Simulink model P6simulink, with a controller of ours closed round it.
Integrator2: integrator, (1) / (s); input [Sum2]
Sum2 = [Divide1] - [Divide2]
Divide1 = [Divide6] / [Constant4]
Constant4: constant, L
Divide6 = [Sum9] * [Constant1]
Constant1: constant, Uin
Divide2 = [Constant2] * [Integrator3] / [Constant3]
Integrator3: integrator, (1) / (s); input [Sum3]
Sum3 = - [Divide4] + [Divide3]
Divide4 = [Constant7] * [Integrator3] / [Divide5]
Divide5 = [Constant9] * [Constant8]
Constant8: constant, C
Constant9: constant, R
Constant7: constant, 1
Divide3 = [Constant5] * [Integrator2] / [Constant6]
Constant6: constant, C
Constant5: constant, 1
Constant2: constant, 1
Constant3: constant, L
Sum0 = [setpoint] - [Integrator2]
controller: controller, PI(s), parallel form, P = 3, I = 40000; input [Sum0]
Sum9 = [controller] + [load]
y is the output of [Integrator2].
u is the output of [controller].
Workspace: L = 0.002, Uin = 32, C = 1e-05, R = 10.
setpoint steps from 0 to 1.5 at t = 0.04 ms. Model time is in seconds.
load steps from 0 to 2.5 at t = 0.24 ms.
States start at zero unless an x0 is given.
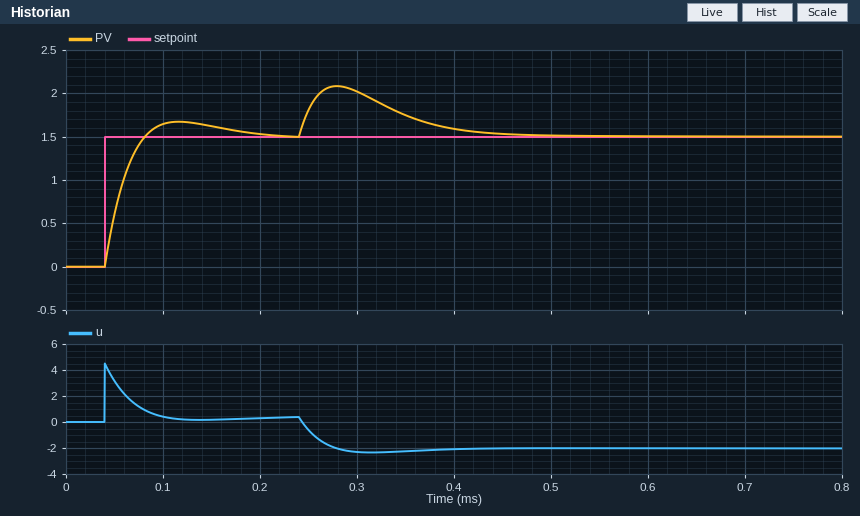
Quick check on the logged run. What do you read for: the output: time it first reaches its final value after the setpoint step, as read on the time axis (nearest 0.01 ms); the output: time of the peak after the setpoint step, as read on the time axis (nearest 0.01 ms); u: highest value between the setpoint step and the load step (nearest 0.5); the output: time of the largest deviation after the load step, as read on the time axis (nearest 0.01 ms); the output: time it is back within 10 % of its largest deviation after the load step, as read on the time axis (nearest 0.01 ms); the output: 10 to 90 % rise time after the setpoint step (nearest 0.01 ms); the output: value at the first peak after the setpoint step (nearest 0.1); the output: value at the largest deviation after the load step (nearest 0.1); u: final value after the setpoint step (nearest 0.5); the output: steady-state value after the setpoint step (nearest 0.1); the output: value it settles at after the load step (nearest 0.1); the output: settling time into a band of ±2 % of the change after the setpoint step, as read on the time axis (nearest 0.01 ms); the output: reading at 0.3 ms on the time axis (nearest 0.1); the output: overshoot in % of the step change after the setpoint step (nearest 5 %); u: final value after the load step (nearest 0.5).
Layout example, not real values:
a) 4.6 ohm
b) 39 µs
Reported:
a) 0.08 ms
b) 0.12 ms
c) 4.5
d) 0.28 ms
e) 0.42 ms
f) 0.03 ms
g) 1.7
h) 2.1
i) 0.5
j) 1.5
k) 1.5
l) 0.20 ms
m) 2.0
n) 10 %
o) -2.0
